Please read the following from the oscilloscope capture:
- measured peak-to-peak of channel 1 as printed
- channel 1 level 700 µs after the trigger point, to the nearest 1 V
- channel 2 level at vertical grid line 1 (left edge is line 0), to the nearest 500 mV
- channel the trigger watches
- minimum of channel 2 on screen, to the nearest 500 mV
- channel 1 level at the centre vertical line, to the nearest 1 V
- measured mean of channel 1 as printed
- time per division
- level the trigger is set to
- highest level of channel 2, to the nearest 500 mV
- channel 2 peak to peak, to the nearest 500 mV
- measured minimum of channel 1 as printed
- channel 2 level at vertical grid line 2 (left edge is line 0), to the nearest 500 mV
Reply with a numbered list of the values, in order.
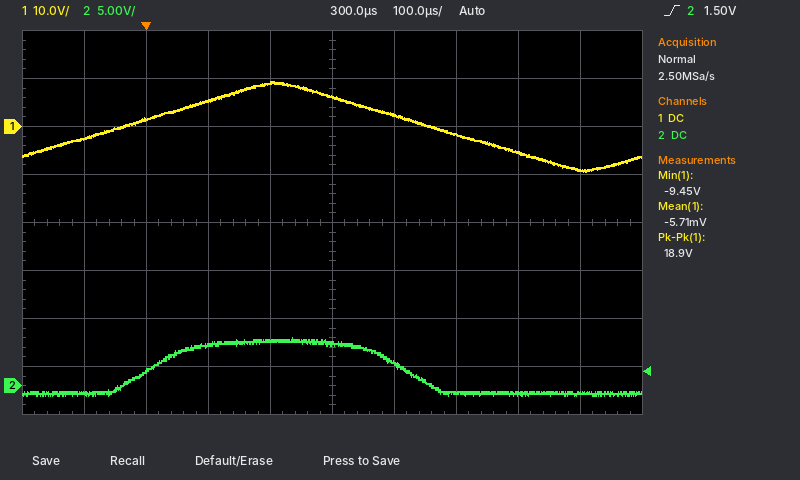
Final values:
1. 18.9 V
2. -9 V
3. -1.0 V
4. channel 2
5. -1.0 V
6. 6 V
7. -5.71 mV
8. 100 µs
9. 1.50 V
10. 5.0 V
11. 6.0 V
12. -9.45 V
13. 1.5 V
